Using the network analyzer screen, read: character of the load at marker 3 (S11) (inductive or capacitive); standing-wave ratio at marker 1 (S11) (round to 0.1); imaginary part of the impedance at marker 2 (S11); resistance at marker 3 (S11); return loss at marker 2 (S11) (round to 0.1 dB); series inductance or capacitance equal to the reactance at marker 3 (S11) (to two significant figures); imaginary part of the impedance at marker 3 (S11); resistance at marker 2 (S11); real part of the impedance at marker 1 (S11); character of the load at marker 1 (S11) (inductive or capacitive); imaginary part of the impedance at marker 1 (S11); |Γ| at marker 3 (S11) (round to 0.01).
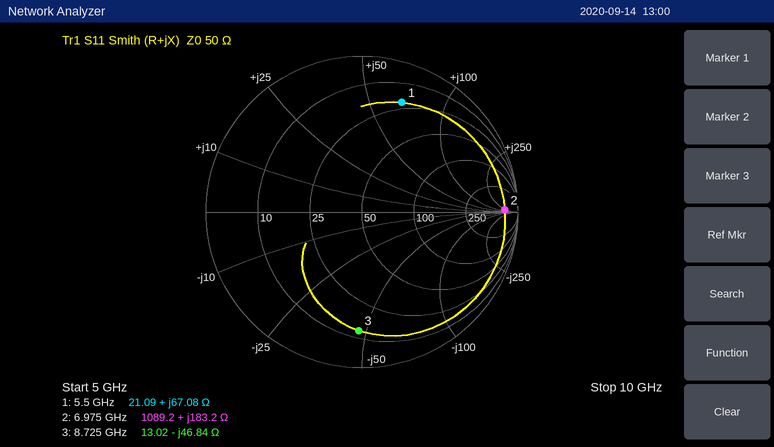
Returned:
capacitive
6.9
+183.2 Ω
13.02 Ω
0.8 dB
390 fF
-46.84 Ω
1089.2 Ω
21.09 Ω
inductive
+67.08 Ω
0.76
